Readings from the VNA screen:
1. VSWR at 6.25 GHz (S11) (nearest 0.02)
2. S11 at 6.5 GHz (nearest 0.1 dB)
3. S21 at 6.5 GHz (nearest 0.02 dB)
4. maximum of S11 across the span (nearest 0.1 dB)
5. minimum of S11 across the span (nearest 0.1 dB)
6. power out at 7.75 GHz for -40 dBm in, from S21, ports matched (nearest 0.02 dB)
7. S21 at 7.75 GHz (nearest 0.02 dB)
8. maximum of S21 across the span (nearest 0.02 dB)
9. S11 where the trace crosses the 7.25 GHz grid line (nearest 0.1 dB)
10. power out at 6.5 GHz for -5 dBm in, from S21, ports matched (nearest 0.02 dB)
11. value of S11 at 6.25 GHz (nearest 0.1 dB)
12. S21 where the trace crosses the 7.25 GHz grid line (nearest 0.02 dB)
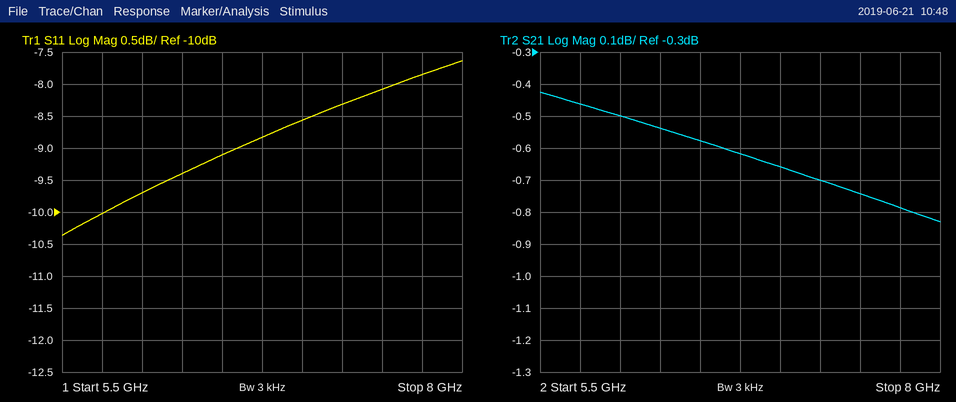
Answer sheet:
2.02
-9.1 dB
-0.58 dB
-7.6 dB
-10.4 dB
-40.78 dBm
-0.78 dB
-0.42 dB
-8.3 dB
-5.58 dBm
-9.4 dB
-0.70 dB
